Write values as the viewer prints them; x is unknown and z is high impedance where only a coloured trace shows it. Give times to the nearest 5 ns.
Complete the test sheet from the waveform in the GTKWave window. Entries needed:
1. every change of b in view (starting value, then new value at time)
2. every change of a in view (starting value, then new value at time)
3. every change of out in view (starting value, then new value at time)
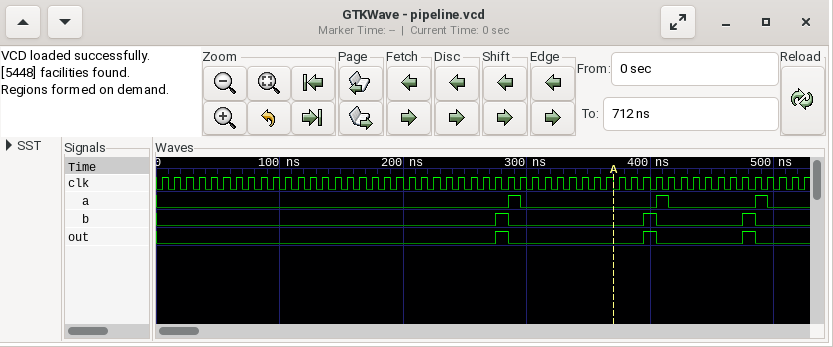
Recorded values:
0, 1 at 275 ns, 0 at 285 ns, 1 at 395 ns, 0 at 405 ns, 1 at 475 ns, 0 at 485 ns
0, 1 at 285 ns, 0 at 295 ns, 1 at 405 ns, 0 at 415 ns, 1 at 485 ns, 0 at 495 ns
0, 1 at 275 ns, 0 at 285 ns, 1 at 395 ns, 0 at 405 ns, 1 at 475 ns, 0 at 485 ns
